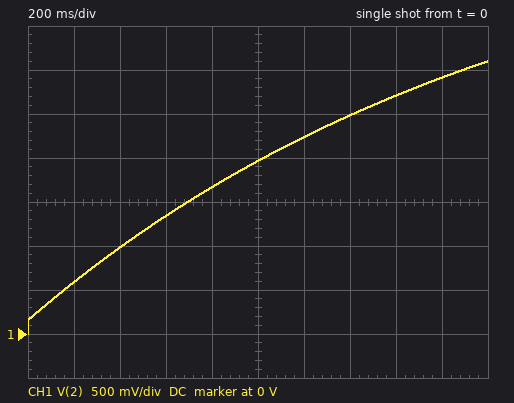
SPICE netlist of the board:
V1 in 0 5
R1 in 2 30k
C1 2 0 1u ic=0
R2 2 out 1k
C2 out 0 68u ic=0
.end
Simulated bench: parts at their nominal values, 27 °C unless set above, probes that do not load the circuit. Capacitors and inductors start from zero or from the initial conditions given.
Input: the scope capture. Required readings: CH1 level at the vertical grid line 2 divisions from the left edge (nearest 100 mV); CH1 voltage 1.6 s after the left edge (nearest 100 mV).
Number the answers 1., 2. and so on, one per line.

1. 1.0 V
2. 2.7 V
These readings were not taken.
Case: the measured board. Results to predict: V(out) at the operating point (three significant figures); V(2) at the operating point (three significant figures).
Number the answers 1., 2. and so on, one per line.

1. 5.00 V
2. 5.00 V
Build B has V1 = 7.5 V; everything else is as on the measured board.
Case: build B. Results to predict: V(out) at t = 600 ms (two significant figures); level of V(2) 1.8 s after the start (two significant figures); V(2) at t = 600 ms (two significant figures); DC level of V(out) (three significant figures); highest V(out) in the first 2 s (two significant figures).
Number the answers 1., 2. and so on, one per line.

1. 1.8 V
2. 4.4 V
3. 2.0 V
4. 7.50 V
5. 4.6 V
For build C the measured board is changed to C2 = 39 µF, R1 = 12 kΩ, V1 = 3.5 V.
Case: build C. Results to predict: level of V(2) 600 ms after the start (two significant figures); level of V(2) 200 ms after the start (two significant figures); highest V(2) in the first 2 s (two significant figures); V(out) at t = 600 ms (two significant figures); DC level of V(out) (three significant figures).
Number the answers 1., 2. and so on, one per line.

1. 2.5 V
2. 1.3 V
3. 3.4 V
4. 2.4 V
5. 3.50 V
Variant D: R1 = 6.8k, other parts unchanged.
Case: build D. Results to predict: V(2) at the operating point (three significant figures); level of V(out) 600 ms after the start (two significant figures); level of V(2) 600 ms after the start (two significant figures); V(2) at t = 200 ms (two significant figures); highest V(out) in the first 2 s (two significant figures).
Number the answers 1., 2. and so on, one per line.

1. 5.00 V
2. 3.4 V
3. 3.6 V
4. 2.0 V
5. 4.9 V
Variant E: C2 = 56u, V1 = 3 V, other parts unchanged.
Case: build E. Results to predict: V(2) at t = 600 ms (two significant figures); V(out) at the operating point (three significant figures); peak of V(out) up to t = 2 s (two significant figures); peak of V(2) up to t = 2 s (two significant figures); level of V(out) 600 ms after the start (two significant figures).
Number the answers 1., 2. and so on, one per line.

1. 930 mV
2. 3.00 V
3. 2.0 V
4. 2.1 V
5. 860 mV
